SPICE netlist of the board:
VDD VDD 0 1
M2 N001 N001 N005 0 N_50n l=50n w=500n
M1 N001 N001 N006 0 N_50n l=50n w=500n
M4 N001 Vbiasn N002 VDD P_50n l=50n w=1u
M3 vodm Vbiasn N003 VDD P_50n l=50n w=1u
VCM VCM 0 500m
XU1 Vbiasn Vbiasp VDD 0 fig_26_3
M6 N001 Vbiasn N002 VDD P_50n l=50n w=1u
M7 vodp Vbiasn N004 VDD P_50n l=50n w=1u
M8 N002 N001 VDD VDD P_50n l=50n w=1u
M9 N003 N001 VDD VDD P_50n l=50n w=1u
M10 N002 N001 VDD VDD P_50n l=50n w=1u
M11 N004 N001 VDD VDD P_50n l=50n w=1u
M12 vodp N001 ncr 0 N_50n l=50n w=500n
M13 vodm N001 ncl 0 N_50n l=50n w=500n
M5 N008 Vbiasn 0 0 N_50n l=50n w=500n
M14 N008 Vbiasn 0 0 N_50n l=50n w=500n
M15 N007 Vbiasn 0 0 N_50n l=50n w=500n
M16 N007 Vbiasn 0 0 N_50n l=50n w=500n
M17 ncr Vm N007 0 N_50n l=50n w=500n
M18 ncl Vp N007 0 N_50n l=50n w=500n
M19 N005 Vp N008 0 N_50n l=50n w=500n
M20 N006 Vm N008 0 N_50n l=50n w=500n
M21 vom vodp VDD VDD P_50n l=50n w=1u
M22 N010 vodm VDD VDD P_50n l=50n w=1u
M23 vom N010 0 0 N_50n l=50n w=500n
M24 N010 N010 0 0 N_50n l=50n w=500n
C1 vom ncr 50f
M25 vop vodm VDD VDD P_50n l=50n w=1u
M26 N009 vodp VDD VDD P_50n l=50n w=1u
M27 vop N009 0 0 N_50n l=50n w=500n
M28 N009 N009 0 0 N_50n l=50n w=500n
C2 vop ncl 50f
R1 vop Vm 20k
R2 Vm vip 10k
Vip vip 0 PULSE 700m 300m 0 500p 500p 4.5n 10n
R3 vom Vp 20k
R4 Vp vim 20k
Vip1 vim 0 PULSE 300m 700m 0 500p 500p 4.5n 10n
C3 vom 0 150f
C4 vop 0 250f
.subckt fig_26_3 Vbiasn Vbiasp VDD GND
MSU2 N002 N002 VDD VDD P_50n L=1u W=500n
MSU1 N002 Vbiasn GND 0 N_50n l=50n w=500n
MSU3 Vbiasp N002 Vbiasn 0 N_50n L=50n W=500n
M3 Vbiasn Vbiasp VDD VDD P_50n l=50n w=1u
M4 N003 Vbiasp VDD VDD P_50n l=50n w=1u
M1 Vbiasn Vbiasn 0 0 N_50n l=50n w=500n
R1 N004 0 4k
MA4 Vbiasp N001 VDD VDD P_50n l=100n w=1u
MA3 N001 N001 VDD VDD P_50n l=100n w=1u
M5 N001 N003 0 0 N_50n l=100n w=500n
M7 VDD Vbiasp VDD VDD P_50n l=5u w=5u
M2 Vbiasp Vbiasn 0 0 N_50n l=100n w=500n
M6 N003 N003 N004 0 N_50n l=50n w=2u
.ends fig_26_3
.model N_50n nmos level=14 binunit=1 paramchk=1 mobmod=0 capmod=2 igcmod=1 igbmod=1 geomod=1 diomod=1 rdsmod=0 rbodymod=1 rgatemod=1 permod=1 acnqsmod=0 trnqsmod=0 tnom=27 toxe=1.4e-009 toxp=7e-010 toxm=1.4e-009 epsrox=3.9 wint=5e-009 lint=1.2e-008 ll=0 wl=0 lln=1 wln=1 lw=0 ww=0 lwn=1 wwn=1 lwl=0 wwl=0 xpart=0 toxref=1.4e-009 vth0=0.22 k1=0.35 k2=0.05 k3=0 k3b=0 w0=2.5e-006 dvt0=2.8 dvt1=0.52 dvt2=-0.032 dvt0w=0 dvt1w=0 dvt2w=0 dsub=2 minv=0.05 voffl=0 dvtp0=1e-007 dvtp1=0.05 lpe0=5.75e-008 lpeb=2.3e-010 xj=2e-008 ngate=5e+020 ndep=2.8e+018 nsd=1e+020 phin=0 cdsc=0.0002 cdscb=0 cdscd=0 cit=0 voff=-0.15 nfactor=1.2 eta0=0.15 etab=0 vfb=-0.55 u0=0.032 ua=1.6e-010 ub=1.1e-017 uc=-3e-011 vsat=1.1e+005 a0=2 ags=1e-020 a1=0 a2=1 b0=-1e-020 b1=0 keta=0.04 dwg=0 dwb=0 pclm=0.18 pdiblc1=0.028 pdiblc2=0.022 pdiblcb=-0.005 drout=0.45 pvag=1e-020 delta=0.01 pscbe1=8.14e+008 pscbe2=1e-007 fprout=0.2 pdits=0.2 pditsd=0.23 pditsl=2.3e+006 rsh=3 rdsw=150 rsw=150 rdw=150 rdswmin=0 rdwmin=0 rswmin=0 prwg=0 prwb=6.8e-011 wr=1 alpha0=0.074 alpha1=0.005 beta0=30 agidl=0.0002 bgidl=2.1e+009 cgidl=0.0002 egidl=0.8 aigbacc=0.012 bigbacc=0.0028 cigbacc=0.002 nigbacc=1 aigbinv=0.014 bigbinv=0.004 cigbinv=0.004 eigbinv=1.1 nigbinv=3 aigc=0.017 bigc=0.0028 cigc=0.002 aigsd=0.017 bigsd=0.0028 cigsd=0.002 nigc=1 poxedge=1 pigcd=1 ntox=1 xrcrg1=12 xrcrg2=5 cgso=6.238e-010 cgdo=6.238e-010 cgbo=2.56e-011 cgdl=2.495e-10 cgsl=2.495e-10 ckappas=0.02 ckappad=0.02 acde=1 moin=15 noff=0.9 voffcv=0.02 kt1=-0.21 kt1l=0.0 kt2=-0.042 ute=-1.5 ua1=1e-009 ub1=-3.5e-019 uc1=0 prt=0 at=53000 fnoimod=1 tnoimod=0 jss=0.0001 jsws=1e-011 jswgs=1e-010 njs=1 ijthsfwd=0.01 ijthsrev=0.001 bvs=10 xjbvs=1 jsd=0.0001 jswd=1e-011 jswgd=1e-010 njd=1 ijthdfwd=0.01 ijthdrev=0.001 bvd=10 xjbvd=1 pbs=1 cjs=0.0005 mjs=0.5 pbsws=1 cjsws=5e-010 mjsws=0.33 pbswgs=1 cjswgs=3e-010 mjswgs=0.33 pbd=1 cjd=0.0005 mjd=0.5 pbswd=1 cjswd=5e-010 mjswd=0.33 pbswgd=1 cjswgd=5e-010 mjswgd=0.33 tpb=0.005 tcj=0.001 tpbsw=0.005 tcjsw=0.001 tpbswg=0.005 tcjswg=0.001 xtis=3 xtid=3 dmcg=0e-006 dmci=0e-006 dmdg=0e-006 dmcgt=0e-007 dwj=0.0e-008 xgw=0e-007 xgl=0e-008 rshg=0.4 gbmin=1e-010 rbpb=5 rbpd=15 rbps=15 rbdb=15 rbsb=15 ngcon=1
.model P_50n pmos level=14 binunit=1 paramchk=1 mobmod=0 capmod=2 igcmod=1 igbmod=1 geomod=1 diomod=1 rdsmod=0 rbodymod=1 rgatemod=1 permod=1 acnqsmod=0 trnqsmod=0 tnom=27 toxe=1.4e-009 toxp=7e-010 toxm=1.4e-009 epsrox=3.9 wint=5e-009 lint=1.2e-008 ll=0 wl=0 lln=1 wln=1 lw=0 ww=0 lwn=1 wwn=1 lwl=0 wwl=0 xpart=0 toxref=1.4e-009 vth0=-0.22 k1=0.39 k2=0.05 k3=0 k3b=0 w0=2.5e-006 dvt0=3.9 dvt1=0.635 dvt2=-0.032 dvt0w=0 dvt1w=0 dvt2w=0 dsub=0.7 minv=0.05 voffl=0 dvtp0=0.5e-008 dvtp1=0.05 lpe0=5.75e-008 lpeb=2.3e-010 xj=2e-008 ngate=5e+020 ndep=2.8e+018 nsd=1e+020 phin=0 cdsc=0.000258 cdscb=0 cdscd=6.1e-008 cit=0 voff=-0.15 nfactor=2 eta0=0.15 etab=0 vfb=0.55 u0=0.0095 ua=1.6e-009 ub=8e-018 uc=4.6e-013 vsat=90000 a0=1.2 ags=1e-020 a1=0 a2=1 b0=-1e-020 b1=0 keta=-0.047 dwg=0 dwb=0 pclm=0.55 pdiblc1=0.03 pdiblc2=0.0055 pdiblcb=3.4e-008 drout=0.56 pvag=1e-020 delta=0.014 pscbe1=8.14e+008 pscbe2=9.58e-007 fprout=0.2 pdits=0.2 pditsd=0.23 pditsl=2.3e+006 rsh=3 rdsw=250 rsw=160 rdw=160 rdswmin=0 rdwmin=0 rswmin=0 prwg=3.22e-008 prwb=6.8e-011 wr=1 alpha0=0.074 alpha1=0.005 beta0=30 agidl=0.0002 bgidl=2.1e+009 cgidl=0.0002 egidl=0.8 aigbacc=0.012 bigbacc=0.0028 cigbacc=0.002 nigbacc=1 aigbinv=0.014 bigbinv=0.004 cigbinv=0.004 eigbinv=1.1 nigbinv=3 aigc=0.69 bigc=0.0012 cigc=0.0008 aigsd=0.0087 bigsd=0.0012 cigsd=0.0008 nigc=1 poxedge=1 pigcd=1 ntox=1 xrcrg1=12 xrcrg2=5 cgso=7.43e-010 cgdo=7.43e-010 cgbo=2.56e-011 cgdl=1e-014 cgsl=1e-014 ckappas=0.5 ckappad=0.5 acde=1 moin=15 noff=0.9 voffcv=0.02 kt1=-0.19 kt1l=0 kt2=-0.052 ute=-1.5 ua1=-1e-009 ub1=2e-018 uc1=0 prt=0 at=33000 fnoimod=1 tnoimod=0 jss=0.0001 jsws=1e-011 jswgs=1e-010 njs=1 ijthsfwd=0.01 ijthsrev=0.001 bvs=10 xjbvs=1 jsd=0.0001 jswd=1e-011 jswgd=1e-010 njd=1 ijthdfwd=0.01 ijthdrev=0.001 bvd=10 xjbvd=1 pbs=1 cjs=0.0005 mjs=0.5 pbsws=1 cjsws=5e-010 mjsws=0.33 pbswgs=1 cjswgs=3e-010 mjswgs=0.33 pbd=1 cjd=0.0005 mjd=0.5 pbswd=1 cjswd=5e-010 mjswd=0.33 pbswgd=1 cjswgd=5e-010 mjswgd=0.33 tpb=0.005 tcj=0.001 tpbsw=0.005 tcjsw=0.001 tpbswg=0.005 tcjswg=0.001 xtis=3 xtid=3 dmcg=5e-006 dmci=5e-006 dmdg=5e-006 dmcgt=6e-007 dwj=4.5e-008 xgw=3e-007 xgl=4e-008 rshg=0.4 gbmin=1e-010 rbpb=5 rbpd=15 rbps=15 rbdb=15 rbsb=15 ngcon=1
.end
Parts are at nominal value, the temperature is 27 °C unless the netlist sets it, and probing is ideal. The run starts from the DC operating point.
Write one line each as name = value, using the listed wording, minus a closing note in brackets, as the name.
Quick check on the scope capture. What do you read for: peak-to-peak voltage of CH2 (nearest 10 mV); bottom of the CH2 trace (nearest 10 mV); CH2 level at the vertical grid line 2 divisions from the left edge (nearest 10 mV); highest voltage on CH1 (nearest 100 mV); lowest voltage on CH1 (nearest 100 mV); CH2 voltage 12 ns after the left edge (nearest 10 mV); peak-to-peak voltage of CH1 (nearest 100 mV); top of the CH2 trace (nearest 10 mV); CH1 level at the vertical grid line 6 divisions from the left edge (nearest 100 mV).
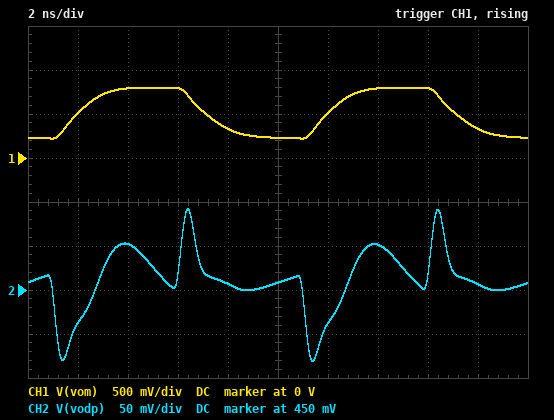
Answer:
peak-to-peak voltage of CH2 = 170 mV
bottom of the CH2 trace = 370 mV
CH2 level at the vertical grid line 2 divisions from the left edge = 500 mV
highest voltage on CH1 = 800 mV
lowest voltage on CH1 = 200 mV
CH2 voltage 12 ns after the left edge = 410 mV
peak-to-peak voltage of CH1 = 600 mV
top of the CH2 trace = 540 mV
CH1 level at the vertical grid line 6 divisions from the left edge = 500 mV
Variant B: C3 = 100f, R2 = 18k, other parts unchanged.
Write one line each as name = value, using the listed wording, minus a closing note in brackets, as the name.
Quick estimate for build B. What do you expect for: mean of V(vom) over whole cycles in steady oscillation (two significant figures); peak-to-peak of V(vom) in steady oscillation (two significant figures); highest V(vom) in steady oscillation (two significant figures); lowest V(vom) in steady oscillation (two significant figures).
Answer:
mean of V(vom) over whole cycles in steady oscillation = 530 mV
peak-to-peak of V(vom) in steady oscillation = 480 mV
highest V(vom) in steady oscillation = 770 mV
lowest V(vom) in steady oscillation = 290 mV
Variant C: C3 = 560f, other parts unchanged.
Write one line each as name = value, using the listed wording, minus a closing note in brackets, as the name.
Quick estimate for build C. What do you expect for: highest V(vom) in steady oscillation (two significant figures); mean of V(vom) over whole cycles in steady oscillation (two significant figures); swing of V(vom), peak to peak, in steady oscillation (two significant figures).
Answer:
highest V(vom) in steady oscillation = 770 mV
mean of V(vom) over whole cycles in steady oscillation = 530 mV
swing of V(vom), peak to peak, in steady oscillation = 510 mV
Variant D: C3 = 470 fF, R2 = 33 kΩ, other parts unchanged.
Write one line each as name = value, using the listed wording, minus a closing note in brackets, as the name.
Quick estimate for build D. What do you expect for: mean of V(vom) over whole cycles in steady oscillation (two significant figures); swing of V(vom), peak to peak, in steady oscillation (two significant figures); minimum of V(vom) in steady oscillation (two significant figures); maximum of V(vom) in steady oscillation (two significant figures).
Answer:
mean of V(vom) over whole cycles in steady oscillation = 530 mV
swing of V(vom), peak to peak, in steady oscillation = 270 mV
minimum of V(vom) in steady oscillation = 390 mV
maximum of V(vom) in steady oscillation = 660 mV
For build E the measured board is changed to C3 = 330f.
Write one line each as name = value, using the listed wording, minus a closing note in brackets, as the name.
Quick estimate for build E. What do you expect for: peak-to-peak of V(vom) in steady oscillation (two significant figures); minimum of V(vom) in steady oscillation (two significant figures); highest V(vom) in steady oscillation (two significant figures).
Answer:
peak-to-peak of V(vom) in steady oscillation = 550 mV
minimum of V(vom) in steady oscillation = 230 mV
highest V(vom) in steady oscillation = 780 mV
